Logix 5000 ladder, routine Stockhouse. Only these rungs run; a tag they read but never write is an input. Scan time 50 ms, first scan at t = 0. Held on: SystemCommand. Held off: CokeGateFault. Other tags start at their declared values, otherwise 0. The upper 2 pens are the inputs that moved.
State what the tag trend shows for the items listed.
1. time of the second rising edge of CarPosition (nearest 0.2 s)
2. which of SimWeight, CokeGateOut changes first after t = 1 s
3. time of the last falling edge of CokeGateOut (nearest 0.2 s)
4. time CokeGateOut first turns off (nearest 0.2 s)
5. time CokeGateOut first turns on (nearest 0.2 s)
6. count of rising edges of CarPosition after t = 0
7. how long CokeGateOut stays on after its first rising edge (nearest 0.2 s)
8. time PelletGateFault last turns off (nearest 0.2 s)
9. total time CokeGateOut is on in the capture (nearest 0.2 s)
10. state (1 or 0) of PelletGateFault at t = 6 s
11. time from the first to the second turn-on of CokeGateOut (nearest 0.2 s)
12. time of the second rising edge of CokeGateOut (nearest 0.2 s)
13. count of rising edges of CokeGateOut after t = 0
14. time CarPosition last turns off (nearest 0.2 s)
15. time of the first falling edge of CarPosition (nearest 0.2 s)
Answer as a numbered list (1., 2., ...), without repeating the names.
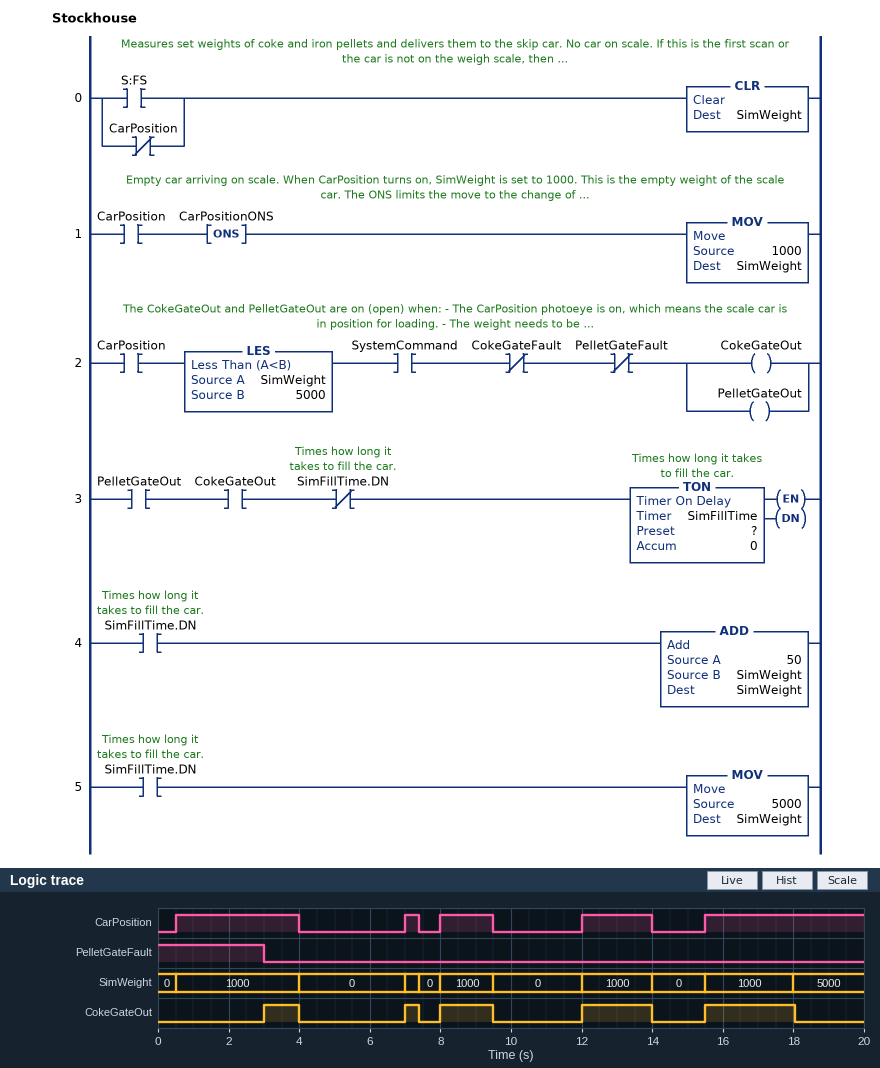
1. 7.0 s
2. CokeGateOut
3. 18.0 s
4. 4.0 s
5. 3.0 s
6. 5
7. 1.0 s
8. 3.0 s
9. 7.4 s
10. 0
11. 4.0 s
12. 7.0 s
13. 5
14. 14.0 s
15. 4.0 s
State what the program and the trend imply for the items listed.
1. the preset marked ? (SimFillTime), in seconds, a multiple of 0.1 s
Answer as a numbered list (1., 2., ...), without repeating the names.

1. 2.5 s
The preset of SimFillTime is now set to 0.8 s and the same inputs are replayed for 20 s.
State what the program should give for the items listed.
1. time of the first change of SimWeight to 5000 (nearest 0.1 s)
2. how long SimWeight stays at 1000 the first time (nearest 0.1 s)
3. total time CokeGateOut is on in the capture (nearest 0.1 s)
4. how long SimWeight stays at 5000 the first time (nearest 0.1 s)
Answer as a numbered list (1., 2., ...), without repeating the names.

1. 3.8 s
2. 3.3 s
3. 3.8 s
4. 0.2 s
